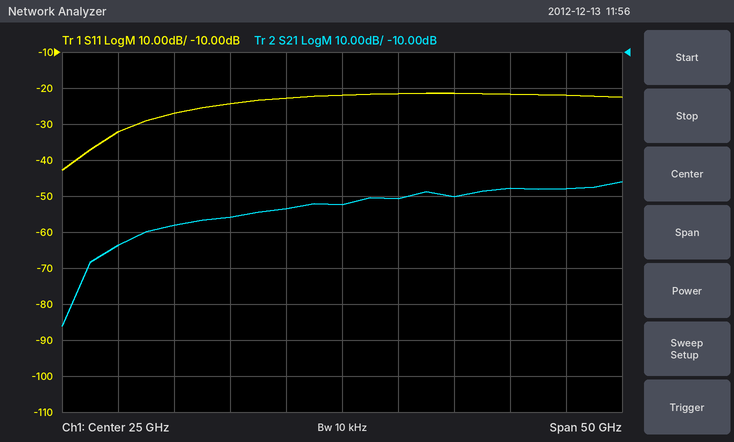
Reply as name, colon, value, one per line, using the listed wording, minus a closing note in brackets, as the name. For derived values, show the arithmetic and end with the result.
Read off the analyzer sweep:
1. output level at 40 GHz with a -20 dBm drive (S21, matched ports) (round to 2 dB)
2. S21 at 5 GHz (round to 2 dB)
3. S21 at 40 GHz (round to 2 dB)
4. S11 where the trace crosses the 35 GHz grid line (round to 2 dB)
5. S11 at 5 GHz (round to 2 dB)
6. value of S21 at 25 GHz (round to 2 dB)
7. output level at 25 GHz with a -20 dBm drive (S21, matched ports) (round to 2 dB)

output level at 40 GHz with a -20 dBm drive (S21, matched ports): -20 dBm + (-48 dB) = -68 dBm
S21 at 5 GHz: -64 dB
S21 at 40 GHz: -48 dB
S11 where the trace crosses the 35 GHz grid line: -22 dB
S11 at 5 GHz: -32 dB
value of S21 at 25 GHz: -52 dB
output level at 25 GHz with a -20 dBm drive (S21, matched ports): -20 dBm + (-52 dB) = -72 dBm
